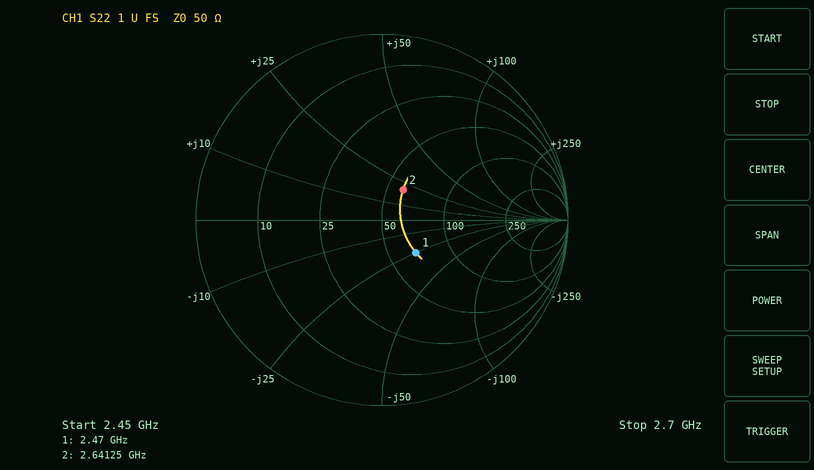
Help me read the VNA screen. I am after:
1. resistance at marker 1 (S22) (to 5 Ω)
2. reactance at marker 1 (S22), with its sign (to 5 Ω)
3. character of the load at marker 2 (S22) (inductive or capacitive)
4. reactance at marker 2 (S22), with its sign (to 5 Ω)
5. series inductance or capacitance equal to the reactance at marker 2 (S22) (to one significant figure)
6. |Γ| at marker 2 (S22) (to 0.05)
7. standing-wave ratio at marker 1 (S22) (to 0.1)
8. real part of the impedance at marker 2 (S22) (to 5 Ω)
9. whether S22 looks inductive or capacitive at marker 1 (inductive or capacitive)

65 Ω
-25 Ω
inductive
+20 Ω
1 nH
0.20
1.7
60 Ω
capacitive
